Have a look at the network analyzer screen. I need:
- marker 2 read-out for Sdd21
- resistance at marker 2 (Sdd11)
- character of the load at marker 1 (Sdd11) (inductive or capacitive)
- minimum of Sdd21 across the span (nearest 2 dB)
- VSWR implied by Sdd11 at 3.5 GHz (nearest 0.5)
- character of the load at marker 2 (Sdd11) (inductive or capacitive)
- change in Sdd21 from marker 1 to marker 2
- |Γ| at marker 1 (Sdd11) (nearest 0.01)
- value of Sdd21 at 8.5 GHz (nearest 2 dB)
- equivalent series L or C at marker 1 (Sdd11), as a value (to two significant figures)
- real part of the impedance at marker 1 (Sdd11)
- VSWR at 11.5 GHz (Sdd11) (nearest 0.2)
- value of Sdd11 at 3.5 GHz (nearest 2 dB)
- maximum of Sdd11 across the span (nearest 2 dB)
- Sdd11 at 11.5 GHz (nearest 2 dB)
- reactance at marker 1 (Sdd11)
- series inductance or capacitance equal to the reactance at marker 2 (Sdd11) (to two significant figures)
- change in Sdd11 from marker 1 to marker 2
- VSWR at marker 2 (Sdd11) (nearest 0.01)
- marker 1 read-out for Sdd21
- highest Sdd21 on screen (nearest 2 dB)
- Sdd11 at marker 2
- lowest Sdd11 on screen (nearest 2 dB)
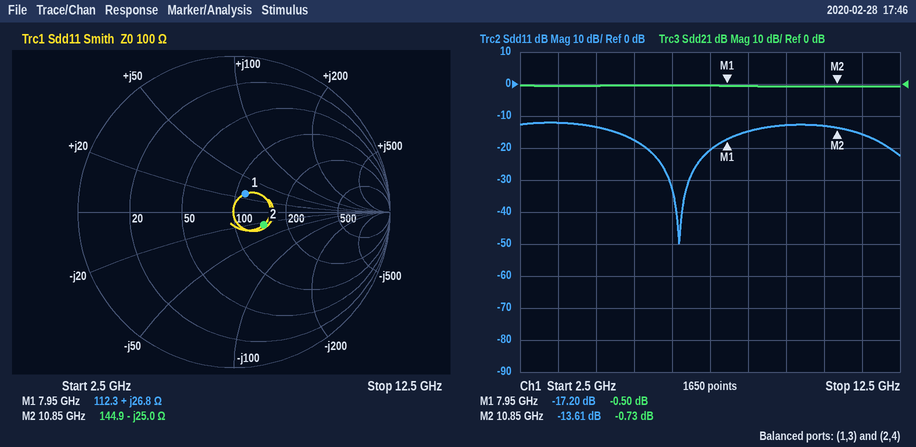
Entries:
-0.73 dB
144.9 Ω
inductive
0 dB
1.5
capacitive
-0.23 dB
0.14
0 dB
540 pH
112.3 Ω
1.4
-12 dB
-12 dB
-16 dB
+26.8 Ω
590 fF
3.59 dB
1.53
-0.50 dB
0 dB
-13.61 dB
-50 dB
